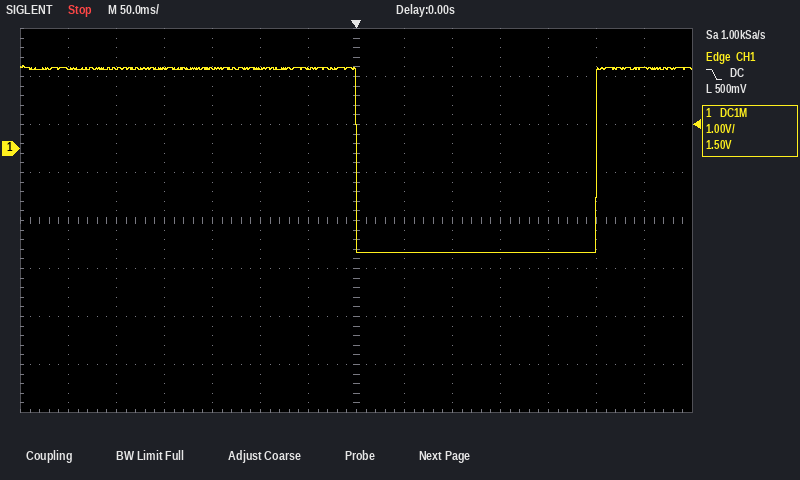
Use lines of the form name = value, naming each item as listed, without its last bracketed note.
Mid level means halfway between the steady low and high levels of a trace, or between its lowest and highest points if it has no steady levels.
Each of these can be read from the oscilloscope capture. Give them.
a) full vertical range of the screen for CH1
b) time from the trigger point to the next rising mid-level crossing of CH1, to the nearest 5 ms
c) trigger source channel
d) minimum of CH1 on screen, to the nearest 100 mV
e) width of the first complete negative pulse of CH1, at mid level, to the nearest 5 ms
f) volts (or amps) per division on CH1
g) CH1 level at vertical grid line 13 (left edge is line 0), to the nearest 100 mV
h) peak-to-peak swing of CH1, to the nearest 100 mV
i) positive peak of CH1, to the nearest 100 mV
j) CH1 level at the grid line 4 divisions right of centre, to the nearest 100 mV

full vertical range of the screen for CH1 = 8 V
time from the trigger point to the next rising mid-level crossing of CH1, to the nearest 5 ms = 250 ms
trigger source channel = CH1
minimum of CH1 on screen, to the nearest 100 mV = -2.2 V
width of the first complete negative pulse of CH1, at mid level, to the nearest 5 ms = 250 ms
volts (or amps) per division on CH1 = 1 V
CH1 level at vertical grid line 13 (left edge is line 0), to the nearest 100 mV = 1.7 V
peak-to-peak swing of CH1, to the nearest 100 mV = 3.9 V
positive peak of CH1, to the nearest 100 mV = 1.7 V
CH1 level at the grid line 4 divisions right of centre, to the nearest 100 mV = -2.2 V
